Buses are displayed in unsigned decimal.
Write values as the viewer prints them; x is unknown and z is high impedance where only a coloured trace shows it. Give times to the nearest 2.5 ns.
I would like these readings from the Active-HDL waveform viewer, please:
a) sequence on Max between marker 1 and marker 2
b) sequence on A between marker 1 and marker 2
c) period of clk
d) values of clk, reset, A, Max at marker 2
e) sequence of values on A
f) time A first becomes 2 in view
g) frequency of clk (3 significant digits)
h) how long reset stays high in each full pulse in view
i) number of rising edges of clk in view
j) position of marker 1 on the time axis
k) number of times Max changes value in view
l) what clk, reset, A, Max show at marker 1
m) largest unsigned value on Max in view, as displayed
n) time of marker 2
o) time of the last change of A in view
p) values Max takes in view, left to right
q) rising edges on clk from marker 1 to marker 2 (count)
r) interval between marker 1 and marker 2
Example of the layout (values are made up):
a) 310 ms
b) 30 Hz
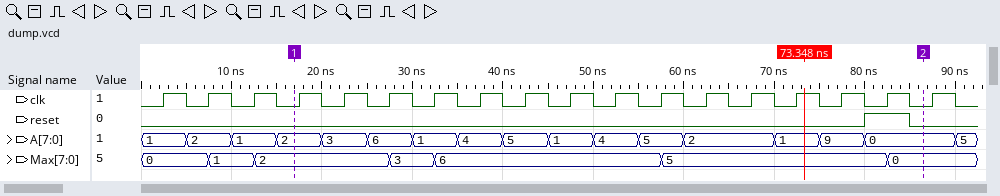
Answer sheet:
a) 2, 3, 6, 5, 0
b) 2, 3, 6, 1, 4, 5, 1, 4, 5, 2, 1, 9, 0
c) 5 ns
d) clk=0, reset=0, A=0, Max=0
e) 1, 2, 1, 2, 3, 6, 1, 4, 5, 1, 4, 5, 2, 1, 9, 0, 5
f) 5 ns
g) 200 MHz
h) 5 ns
i) 18
j) 17.5 ns
k) 6
l) clk=0, reset=0, A=2, Max=2
m) 6
n) 87.5 ns
o) 90 ns
p) 0, 1, 2, 3, 6, 5, 0
q) 14
r) 70 ns
